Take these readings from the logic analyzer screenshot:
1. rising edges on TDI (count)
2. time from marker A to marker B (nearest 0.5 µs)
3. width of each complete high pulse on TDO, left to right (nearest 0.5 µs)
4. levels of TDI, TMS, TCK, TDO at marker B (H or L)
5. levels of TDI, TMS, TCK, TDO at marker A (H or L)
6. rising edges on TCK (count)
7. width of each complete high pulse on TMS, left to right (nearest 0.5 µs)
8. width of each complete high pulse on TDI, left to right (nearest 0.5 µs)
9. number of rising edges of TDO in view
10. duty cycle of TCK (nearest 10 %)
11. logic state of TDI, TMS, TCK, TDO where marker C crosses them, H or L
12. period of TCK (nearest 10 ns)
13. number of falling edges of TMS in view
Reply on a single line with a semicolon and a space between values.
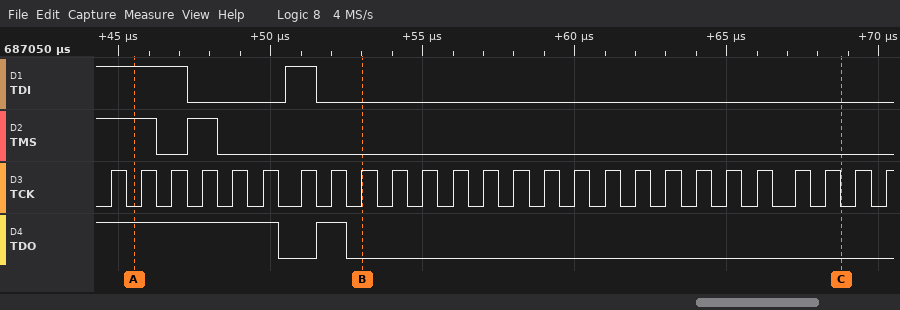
1; 7.5 µs; 1 µs; TDI=L, TMS=L, TCK=H, TDO=L; TDI=H, TMS=H, TCK=L, TDO=H; 26; 1 µs; 1 µs; 1; 50 %; TDI=L, TMS=L, TCK=L, TDO=L; 1020 ns; 2
